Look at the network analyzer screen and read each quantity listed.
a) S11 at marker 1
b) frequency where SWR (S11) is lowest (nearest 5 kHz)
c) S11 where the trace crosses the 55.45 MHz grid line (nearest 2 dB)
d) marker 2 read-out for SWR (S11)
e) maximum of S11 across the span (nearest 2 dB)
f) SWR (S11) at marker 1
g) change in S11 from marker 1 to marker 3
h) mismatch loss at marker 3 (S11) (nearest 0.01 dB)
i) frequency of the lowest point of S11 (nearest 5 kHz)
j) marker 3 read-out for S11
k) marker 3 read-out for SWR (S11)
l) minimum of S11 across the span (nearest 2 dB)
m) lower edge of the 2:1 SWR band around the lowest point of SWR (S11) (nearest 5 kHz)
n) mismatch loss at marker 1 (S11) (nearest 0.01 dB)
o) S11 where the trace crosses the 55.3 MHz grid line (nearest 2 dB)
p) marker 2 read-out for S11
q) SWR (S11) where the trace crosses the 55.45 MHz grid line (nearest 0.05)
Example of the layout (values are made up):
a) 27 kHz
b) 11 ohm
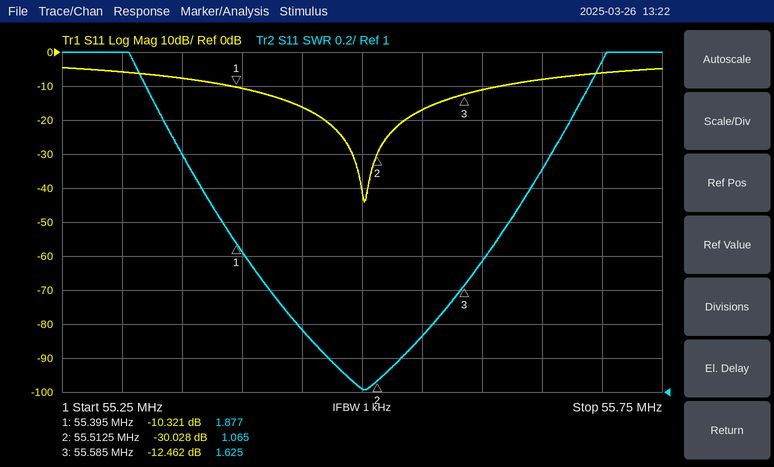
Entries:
a) -10.321 dB
b) 55.500 MHz
c) -16 dB
d) 1.065
e) -4 dB
f) 1.877
g) -2.141 dB
h) 0.25 dB
i) 55.500 MHz
j) -12.462 dB
k) 1.625
l) -44 dB
m) 55.385 MHz
n) 0.42 dB
o) -6 dB
p) -30.028 dB
q) 1.35
